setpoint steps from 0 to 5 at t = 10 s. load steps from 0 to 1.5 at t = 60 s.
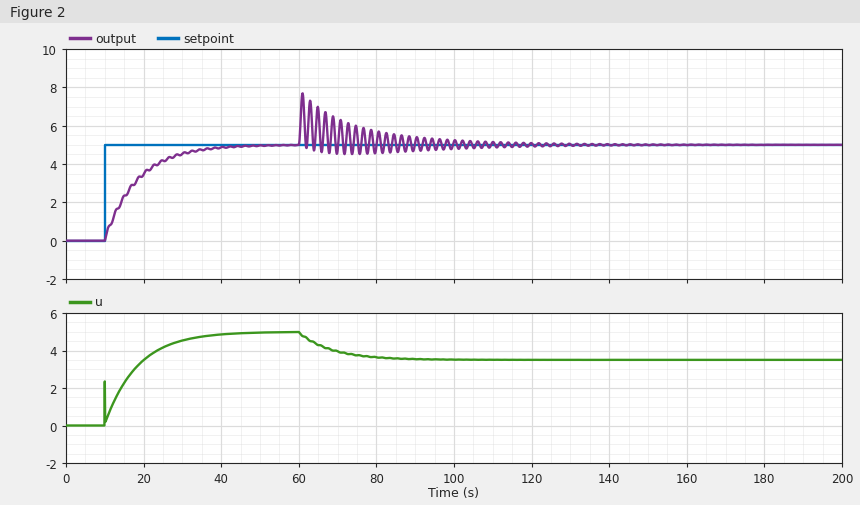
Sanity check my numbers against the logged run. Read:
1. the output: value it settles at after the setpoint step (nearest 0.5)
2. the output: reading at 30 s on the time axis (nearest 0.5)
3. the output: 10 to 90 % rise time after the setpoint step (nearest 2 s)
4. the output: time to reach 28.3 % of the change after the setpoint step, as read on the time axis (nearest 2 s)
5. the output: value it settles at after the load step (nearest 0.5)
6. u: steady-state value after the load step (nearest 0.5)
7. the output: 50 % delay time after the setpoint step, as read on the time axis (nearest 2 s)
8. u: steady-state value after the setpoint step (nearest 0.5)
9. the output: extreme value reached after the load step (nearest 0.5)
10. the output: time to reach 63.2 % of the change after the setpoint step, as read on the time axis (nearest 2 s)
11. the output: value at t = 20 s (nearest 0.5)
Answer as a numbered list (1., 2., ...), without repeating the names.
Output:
1. 5.0
2. 4.5
3. 18 s
4. 12 s
5. 5.0
6. 3.5
7. 16 s
8. 5.0
9. 7.5
10. 18 s
11. 3.5
